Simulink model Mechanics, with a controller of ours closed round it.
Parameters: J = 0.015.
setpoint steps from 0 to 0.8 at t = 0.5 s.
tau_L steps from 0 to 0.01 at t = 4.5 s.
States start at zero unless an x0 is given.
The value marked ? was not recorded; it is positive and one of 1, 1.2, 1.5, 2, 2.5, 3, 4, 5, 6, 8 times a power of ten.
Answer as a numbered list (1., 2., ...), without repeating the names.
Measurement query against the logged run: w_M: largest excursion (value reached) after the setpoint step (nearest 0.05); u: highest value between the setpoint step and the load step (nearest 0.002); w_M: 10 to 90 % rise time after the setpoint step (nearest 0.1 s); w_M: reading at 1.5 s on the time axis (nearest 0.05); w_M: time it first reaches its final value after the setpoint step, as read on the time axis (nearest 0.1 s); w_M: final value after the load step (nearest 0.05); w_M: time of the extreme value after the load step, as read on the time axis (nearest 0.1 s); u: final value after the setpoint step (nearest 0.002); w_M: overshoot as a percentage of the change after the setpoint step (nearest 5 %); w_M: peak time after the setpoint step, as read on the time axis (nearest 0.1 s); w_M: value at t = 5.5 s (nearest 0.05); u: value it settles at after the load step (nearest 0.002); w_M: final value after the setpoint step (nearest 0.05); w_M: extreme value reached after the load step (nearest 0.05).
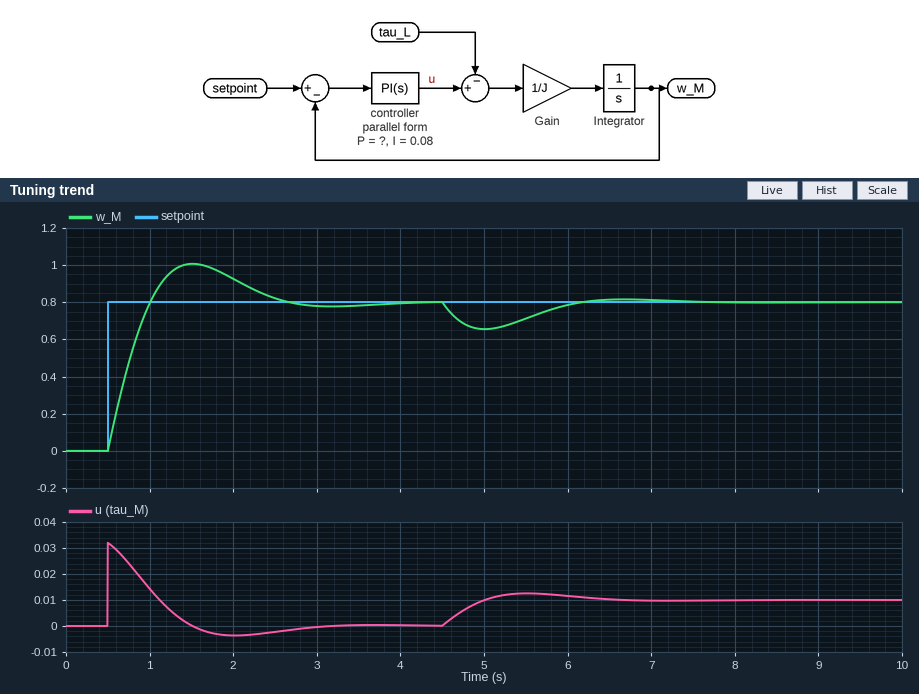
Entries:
1. 1.00
2. 0.032
3. 0.4 s
4. 1.00
5. 1.0 s
6. 0.80
7. 5.0 s
8. 0.000
9. 25 %
10. 1.5 s
11. 0.70
12. 0.010
13. 0.80
14. 0.65
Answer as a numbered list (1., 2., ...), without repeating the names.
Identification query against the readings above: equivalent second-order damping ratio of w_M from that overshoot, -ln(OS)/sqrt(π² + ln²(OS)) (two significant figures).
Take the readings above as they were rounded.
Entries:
1. 0.40
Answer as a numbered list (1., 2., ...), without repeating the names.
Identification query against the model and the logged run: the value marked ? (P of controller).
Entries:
1. 0.04
